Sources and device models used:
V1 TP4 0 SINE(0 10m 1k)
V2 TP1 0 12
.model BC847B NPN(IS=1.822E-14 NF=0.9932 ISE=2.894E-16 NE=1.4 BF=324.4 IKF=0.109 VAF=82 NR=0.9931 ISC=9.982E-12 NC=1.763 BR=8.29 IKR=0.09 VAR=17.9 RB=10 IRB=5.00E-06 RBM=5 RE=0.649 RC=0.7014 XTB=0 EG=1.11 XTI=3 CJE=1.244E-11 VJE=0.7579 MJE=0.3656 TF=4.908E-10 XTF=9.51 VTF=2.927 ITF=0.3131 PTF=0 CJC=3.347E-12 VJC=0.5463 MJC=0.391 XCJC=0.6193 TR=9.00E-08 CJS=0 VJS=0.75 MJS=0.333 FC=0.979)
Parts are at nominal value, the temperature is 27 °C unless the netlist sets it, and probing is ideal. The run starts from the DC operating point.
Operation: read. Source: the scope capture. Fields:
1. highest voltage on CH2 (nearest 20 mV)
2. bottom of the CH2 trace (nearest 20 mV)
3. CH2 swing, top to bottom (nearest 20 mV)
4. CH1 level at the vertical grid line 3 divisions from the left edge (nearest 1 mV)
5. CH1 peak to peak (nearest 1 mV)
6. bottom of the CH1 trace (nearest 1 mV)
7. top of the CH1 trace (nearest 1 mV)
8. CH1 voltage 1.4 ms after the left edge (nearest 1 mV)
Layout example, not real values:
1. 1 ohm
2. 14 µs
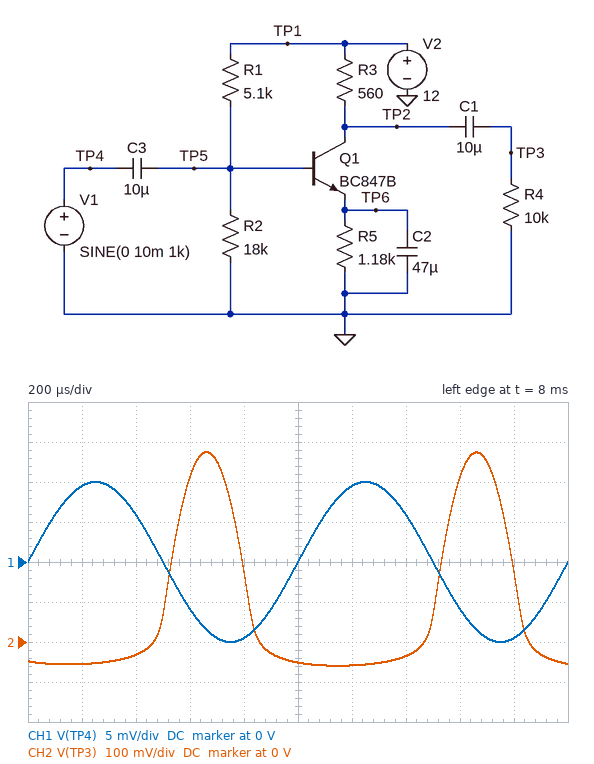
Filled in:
1. 480 mV
2. -60 mV
3. 540 mV
4. -6 mV
5. 20 mV
6. -10 mV
7. 10 mV
8. 6 mV
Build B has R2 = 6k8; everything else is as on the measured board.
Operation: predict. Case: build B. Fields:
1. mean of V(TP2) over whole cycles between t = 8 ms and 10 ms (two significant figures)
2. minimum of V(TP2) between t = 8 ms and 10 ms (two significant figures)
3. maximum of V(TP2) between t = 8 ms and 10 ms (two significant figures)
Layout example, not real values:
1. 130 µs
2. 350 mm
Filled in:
1. 9.1 V
2. 8.3 V
3. 9.8 V
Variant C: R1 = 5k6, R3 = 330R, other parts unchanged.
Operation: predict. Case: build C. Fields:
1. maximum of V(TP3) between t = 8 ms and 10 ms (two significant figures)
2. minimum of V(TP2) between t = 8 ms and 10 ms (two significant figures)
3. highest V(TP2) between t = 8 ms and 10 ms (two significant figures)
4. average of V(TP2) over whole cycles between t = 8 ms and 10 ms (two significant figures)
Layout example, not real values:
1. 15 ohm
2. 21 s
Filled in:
1. 520 mV
2. 9.1 V
3. 10 V
4. 9.7 V
